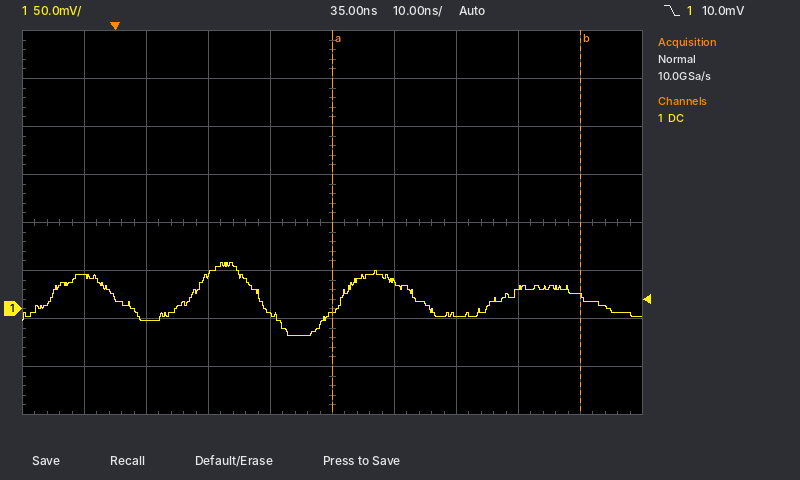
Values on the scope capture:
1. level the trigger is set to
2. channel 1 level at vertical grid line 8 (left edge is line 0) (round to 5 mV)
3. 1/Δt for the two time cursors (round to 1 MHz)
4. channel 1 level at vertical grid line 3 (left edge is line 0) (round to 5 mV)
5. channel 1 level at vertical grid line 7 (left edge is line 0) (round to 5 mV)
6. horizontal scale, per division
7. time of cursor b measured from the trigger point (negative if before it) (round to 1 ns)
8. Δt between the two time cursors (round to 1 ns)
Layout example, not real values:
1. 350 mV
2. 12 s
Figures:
1. 10.0 mV
2. 20 mV
3. 25 MHz
4. 35 mV
5. -5 mV
6. 10 ns
7. +75 ns
8. 40 ns
